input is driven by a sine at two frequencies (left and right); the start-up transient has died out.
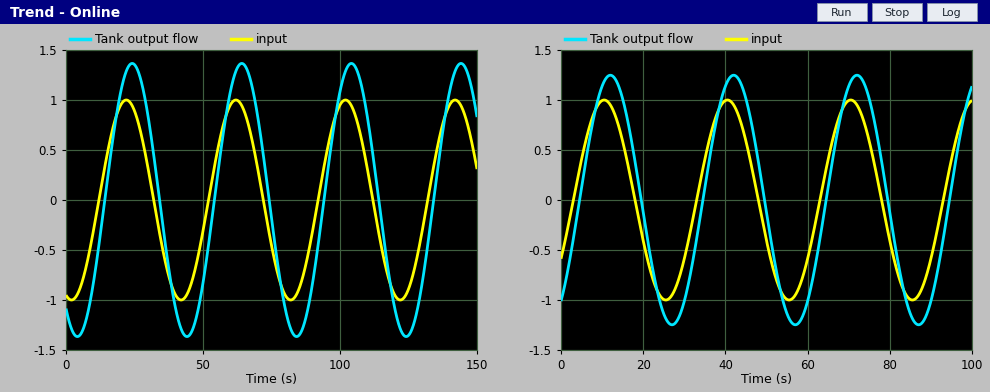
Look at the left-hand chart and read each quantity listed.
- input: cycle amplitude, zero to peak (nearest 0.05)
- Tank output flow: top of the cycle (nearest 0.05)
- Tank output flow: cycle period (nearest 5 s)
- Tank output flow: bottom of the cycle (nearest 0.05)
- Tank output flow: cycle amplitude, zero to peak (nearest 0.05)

1.00
1.35
40 s
-1.35
1.35
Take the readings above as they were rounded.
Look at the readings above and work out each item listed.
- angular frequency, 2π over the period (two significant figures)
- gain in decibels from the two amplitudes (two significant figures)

0.16 rad/s
2.6 dB
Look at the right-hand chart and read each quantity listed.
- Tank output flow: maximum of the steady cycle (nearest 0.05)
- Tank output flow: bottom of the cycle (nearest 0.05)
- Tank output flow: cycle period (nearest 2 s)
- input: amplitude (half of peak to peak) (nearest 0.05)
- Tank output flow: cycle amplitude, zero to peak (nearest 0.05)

1.25
-1.25
30 s
1.00
1.25
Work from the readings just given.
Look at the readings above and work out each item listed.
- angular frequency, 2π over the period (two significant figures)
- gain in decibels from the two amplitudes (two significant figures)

0.21 rad/s
1.9 dB
